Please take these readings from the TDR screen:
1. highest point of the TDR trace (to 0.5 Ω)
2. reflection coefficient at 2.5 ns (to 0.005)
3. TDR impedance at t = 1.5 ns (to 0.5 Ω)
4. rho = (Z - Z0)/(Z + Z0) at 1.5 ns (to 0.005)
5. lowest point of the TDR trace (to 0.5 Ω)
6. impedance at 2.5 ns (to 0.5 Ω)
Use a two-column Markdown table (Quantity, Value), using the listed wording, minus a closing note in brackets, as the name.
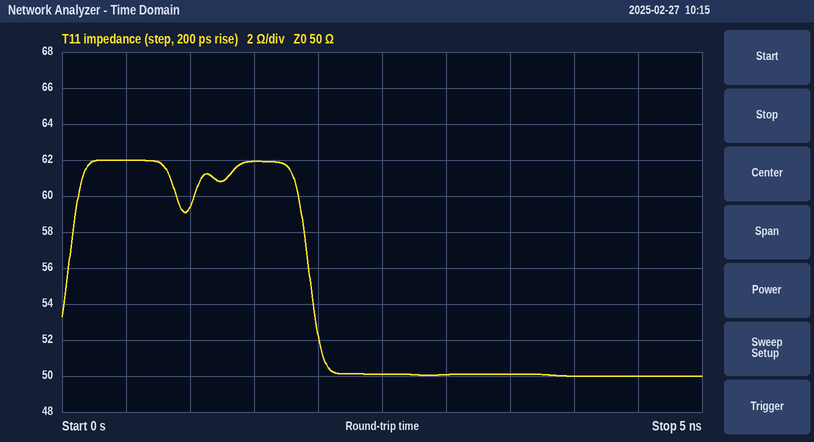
| Quantity | Value |
|---|---|
| highest point of the TDR trace | 62.0 Ω |
| reflection coefficient at 2.5 ns | 0.000 |
| TDR impedance at t = 1.5 ns | 62.0 Ω |
| rho = (Z - Z0)/(Z + Z0) at 1.5 ns | +0.105 |
| lowest point of the TDR trace | 50.0 Ω |
| impedance at 2.5 ns | 50.0 Ω |
